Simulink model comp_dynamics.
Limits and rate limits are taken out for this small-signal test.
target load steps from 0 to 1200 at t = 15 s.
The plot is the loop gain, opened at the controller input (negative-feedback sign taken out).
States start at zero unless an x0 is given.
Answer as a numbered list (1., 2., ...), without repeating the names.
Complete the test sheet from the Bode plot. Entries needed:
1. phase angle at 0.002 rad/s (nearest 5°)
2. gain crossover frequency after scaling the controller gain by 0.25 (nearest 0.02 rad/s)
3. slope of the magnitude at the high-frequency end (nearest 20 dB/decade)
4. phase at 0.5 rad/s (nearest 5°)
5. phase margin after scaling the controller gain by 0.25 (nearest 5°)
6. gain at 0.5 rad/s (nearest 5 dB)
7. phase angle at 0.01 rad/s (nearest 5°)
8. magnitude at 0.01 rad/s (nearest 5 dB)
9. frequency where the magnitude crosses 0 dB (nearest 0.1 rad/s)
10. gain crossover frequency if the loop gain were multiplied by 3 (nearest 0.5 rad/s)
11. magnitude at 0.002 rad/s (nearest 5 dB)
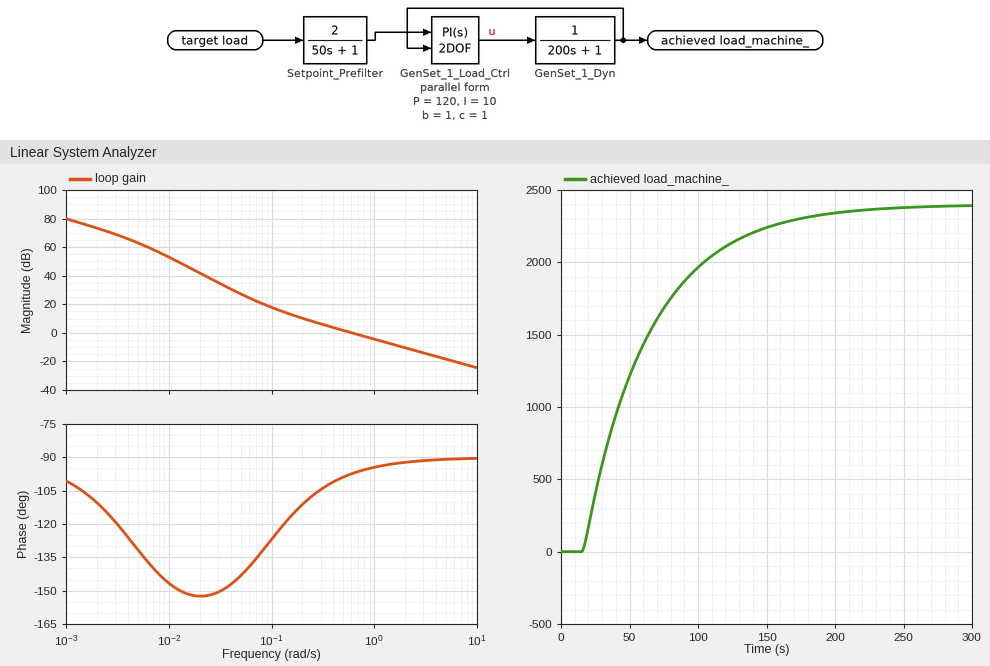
1. -110°
2. 0.16 rad/s
3. -20 dB/decade
4. -100°
5. 65°
6. 0 dB
7. -145°
8. 55 dB
9. 0.6 rad/s
10. 2.0 rad/s
11. 75 dB
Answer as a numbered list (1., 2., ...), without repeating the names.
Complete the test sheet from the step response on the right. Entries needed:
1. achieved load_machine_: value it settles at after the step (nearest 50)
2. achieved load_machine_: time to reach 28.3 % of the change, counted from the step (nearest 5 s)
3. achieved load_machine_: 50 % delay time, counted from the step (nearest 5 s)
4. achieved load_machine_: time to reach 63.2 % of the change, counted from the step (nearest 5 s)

1. 2400
2. 15 s
3. 35 s
4. 50 s
